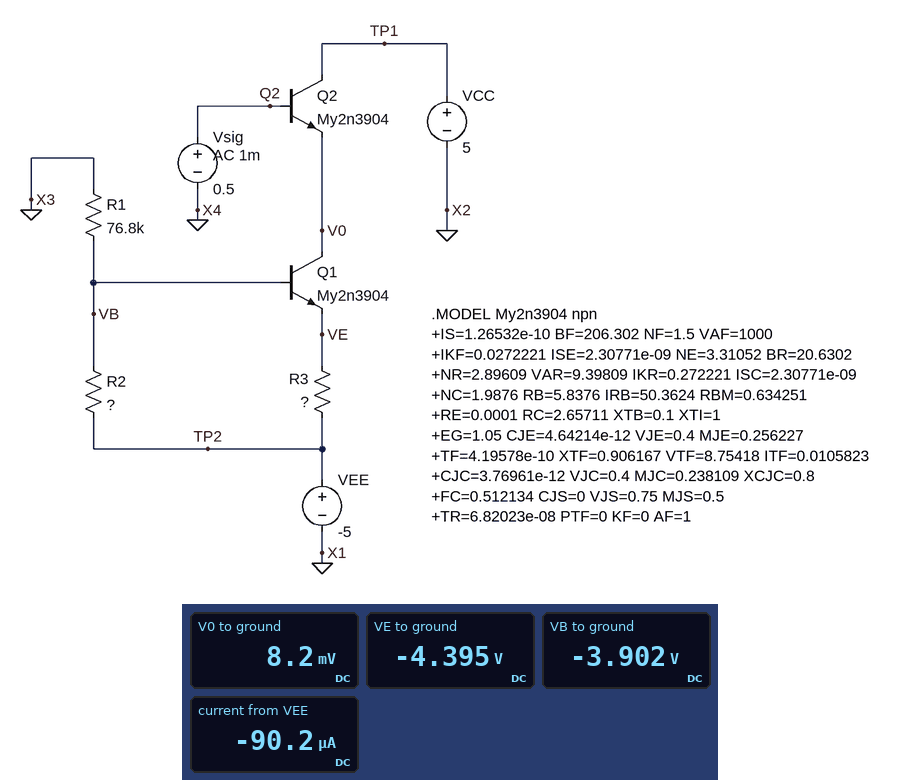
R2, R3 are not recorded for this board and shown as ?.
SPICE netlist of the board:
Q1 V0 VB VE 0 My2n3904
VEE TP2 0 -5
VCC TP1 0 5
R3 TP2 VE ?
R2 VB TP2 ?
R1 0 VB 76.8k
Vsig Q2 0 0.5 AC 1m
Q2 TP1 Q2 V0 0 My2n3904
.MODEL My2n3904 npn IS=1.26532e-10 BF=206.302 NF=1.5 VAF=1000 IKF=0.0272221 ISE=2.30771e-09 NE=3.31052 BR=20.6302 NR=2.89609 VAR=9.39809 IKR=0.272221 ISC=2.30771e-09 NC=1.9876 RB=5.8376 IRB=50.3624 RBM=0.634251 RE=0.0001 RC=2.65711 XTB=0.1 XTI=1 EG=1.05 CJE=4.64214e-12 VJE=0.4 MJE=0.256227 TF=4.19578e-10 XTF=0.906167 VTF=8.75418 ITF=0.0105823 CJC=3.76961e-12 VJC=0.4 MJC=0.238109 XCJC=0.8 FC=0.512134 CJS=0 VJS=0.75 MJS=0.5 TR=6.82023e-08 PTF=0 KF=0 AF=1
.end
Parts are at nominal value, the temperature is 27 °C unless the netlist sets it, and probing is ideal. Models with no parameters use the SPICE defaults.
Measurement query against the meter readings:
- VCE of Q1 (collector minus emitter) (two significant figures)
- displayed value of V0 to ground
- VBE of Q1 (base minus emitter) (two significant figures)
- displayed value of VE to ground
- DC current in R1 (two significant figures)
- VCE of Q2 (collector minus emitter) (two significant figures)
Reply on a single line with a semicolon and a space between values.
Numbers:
4.4 V; 8.2 mV; 490 mV; -4.395 V; 51 µA; 5.0 V
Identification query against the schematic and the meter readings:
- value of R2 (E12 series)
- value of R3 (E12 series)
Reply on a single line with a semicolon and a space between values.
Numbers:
22 kΩ; 15 kΩ
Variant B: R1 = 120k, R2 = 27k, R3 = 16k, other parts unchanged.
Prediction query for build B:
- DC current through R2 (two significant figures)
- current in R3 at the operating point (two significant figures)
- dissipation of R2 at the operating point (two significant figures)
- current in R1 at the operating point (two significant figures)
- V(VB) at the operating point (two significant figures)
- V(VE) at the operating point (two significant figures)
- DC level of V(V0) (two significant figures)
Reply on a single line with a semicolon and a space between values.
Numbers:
33 µA; 27 µA; 30 µW; 34 µA; -4.1 V; -4.6 V; 25 mV
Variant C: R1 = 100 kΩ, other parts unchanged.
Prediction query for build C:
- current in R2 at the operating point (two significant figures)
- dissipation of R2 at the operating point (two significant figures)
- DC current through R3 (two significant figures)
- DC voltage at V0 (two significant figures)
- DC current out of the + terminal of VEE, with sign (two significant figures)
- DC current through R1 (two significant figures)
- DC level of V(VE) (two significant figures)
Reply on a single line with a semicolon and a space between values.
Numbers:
40 µA; 36 µW; 27 µA; 24 mV; -68 µA; 41 µA; -4.6 V
